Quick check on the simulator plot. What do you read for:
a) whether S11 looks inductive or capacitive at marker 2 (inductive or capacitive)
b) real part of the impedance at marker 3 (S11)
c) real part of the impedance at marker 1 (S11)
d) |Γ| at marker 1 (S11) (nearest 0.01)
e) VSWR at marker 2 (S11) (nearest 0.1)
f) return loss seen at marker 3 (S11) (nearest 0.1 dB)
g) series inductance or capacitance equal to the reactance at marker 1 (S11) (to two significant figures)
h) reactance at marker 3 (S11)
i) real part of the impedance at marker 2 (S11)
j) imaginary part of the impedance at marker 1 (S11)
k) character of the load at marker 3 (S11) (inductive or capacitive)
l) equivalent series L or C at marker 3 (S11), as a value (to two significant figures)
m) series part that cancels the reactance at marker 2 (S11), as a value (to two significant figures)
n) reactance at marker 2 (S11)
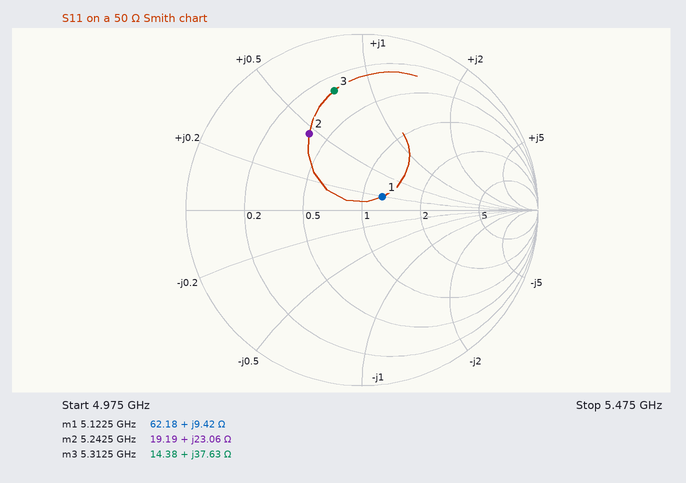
inductive
14.38 Ω
62.18 Ω
0.14
3.2
3.2 dB
290 pH
+37.63 Ω
19.19 Ω
+9.42 Ω
inductive
1.1 nH
1.3 pF
+23.06 Ω
